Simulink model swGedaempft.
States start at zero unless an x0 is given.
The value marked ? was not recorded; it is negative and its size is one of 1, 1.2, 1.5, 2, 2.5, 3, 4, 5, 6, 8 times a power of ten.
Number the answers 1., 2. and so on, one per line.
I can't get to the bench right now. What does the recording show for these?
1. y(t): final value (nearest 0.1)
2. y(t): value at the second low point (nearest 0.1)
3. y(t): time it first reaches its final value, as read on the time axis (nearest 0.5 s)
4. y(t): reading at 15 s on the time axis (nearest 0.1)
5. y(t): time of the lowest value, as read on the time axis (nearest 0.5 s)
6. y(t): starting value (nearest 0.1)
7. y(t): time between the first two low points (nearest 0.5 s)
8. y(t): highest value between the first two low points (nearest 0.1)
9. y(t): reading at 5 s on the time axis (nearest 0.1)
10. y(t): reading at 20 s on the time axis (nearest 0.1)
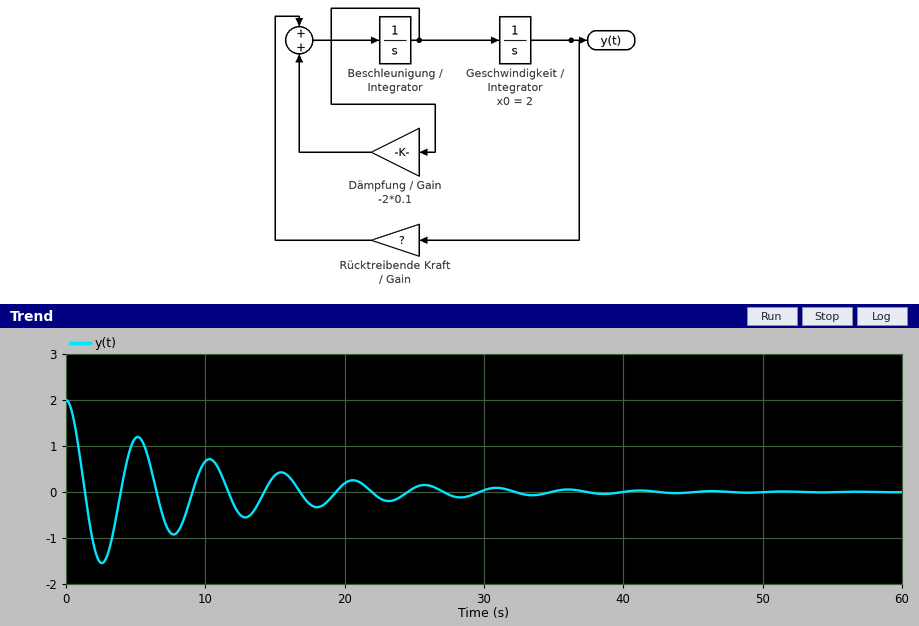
1. 0.0
2. -0.9
3. 1.5 s
4. 0.4
5. 2.5 s
6. 2.0
7. 5.0 s
8. 1.2
9. 1.2
10. 0.2
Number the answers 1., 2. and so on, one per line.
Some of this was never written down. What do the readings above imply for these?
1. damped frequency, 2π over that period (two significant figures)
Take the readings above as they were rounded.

1. 1.3 rad/s
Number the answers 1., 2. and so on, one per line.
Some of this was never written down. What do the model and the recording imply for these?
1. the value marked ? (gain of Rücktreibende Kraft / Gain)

1. -1.5
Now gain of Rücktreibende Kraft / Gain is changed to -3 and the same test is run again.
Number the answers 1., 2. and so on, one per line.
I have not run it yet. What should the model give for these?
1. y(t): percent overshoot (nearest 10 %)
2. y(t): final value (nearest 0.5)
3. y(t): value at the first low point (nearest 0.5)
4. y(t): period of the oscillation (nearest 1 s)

1. 80 %
2. 0.0
3. -1.5
4. 4 s
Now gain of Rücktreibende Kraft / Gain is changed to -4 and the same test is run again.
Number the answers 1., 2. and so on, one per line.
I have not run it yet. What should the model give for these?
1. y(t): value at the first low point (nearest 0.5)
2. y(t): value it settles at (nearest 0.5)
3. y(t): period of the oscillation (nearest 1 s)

1. -1.5
2. 0.0
3. 3 s
